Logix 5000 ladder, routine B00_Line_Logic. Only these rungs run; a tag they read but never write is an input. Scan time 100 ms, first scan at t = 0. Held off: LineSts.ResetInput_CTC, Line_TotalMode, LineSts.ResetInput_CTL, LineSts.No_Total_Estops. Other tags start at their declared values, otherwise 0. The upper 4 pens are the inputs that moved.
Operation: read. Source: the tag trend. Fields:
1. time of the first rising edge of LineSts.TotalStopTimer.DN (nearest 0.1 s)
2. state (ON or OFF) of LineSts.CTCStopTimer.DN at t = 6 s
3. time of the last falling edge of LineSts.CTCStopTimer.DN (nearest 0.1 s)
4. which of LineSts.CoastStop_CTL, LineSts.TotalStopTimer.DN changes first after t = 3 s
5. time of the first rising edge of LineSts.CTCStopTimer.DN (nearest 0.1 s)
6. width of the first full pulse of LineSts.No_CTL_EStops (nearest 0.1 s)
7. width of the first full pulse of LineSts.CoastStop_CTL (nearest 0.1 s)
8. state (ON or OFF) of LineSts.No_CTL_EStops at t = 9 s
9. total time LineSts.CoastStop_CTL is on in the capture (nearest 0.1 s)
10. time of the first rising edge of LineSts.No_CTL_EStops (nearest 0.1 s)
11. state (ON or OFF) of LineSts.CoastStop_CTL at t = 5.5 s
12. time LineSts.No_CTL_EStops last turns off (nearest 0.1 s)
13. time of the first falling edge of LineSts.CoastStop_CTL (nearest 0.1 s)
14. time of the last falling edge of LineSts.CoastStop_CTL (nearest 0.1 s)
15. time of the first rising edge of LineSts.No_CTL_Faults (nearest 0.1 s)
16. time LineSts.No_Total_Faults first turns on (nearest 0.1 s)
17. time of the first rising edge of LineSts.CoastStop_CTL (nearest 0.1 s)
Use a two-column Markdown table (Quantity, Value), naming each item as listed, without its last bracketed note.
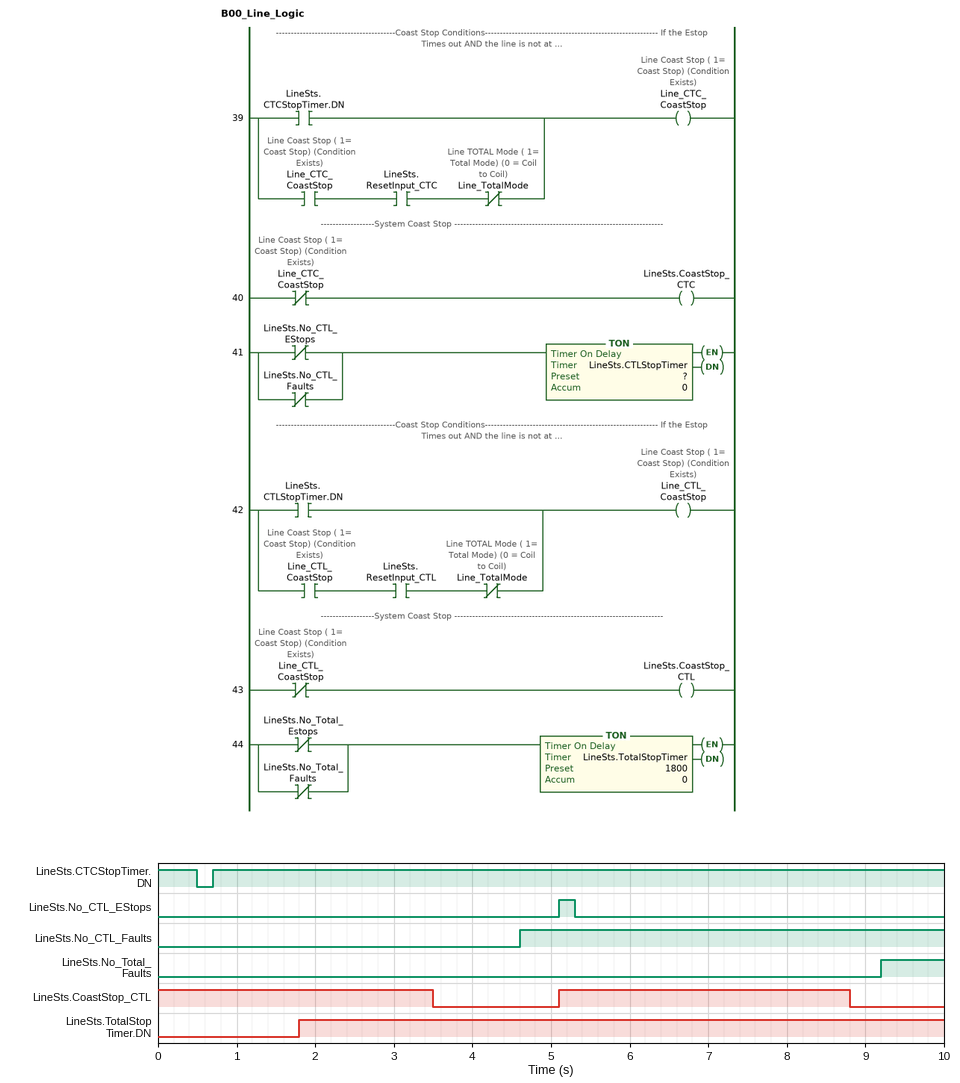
| Quantity | Value |
|---|---|
| time of the first rising edge of LineSts.TotalStopTimer.DN | 1.8 s |
| state (ON or OFF) of LineSts.CTCStopTimer.DN at t = 6 s | ON |
| time of the last falling edge of LineSts.CTCStopTimer.DN | 0.5 s |
| which of LineSts.CoastStop_CTL, LineSts.TotalStopTimer.DN changes first after t = 3 s | LineSts.CoastStop_CTL |
| time of the first rising edge of LineSts.CTCStopTimer.DN | 0.7 s |
| width of the first full pulse of LineSts.No_CTL_EStops | 0.2 s |
| width of the first full pulse of LineSts.CoastStop_CTL | 3.7 s |
| state (ON or OFF) of LineSts.No_CTL_EStops at t = 9 s | OFF |
| total time LineSts.CoastStop_CTL is on in the capture | 7.2 s |
| time of the first rising edge of LineSts.No_CTL_EStops | 5.1 s |
| state (ON or OFF) of LineSts.CoastStop_CTL at t = 5.5 s | ON |
| time LineSts.No_CTL_EStops last turns off | 5.3 s |
| time of the first falling edge of LineSts.CoastStop_CTL | 3.5 s |
| time of the last falling edge of LineSts.CoastStop_CTL | 8.8 s |
| time of the first rising edge of LineSts.No_CTL_Faults | 4.6 s |
| time LineSts.No_Total_Faults first turns on | 9.2 s |
| time of the first rising edge of LineSts.CoastStop_CTL | 5.1 s |
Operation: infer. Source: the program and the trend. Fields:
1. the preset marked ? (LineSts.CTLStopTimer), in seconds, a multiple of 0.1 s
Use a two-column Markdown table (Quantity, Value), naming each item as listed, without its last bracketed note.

| Quantity | Value |
|---|---|
| the preset marked ? (LineSts.CTLStopTimer), in seconds, a multiple of 0.1 s | 3.5 s |
